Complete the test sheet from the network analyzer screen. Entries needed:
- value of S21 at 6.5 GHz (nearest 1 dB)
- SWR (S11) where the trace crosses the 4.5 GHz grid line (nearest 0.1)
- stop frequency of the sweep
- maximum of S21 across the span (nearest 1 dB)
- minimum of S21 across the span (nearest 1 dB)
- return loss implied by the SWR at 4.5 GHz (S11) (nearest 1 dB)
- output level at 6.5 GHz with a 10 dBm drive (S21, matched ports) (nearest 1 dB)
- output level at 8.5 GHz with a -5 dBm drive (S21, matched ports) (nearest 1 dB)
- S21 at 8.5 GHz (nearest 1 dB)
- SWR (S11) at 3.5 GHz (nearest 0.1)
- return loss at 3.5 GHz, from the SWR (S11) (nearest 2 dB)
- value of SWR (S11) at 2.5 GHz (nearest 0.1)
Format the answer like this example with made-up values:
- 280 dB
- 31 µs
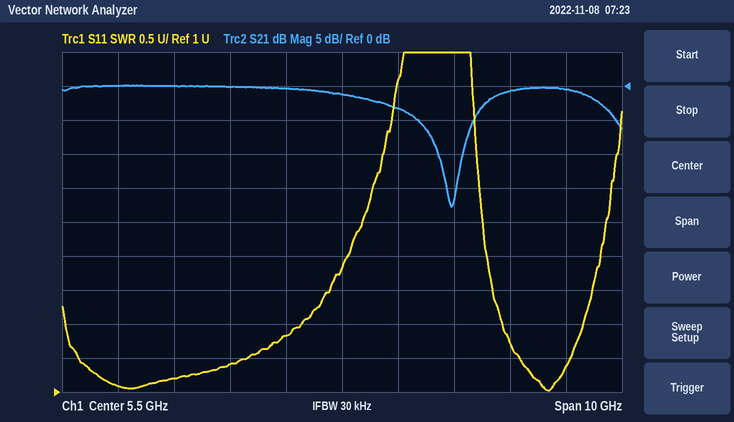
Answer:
- -3 dB
- 1.8
- 10.5 GHz
- 0 dB
- -18 dB
- 11 dB
- 7 dBm
- -6 dBm
- -1 dB
- 1.4
- 16 dB
- 1.2
